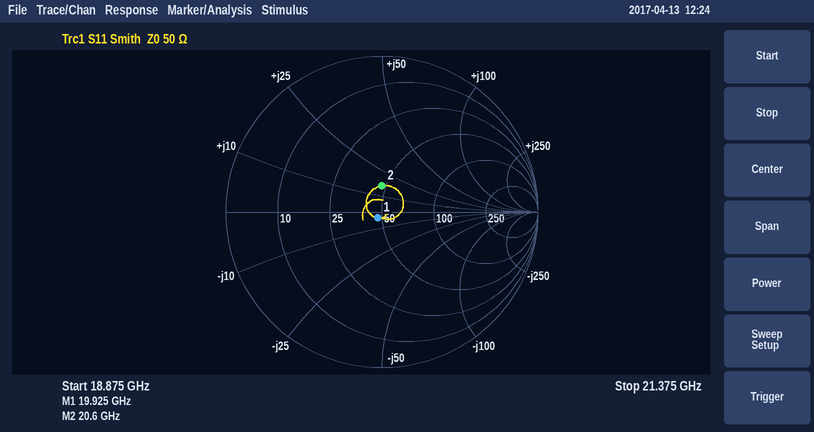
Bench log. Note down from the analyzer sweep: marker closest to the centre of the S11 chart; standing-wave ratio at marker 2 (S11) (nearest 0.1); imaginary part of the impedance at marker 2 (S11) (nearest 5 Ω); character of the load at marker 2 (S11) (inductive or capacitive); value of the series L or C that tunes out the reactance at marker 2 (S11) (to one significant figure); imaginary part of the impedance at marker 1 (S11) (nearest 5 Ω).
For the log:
marker 1
1.4
+15 Ω
inductive
500 fF
-5 Ω
